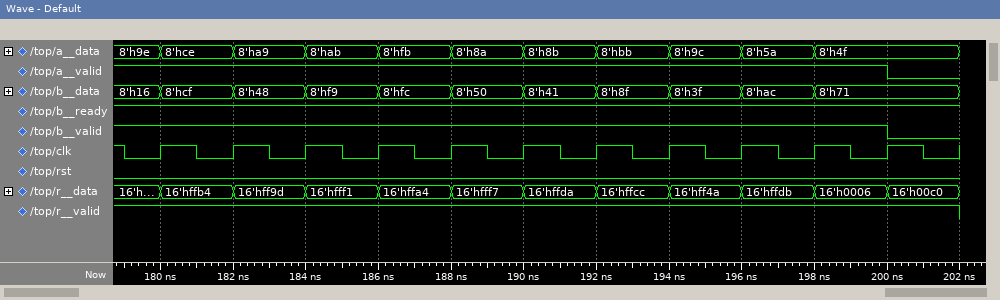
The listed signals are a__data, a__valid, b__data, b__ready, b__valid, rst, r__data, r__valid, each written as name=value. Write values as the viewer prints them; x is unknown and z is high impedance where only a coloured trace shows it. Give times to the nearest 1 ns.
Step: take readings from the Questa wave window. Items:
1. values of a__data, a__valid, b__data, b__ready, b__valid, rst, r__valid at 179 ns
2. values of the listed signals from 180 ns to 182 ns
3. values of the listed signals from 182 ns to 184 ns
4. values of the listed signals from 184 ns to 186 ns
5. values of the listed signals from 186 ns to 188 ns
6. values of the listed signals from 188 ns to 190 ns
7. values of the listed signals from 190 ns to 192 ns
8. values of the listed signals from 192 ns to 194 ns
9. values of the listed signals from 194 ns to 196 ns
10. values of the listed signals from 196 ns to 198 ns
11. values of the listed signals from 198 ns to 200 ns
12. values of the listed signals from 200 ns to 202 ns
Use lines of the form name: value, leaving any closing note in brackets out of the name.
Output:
values of a__data, a__valid, b__data, b__ready, b__valid, rst, r__valid at 179 ns: a__data=8'h9e, a__valid=1, b__data=8'h16, b__ready=1, b__valid=1, rst=0, r__valid=1
values of the listed signals from 180 ns to 182 ns: a__data=8'hce, a__valid=1, b__data=8'hcf, b__ready=1, b__valid=1, rst=0, r__data=16'hffb4, r__valid=1
values of the listed signals from 182 ns to 184 ns: a__data=8'ha9, a__valid=1, b__data=8'h48, b__ready=1, b__valid=1, rst=0, r__data=16'hff9d, r__valid=1
values of the listed signals from 184 ns to 186 ns: a__data=8'hab, a__valid=1, b__data=8'hf9, b__ready=1, b__valid=1, rst=0, r__data=16'hfff1, r__valid=1
values of the listed signals from 186 ns to 188 ns: a__data=8'hfb, a__valid=1, b__data=8'hfc, b__ready=1, b__valid=1, rst=0, r__data=16'hffa4, r__valid=1
values of the listed signals from 188 ns to 190 ns: a__data=8'h8a, a__valid=1, b__data=8'h50, b__ready=1, b__valid=1, rst=0, r__data=16'hfff7, r__valid=1
values of the listed signals from 190 ns to 192 ns: a__data=8'h8b, a__valid=1, b__data=8'h41, b__ready=1, b__valid=1, rst=0, r__data=16'hffda, r__valid=1
values of the listed signals from 192 ns to 194 ns: a__data=8'hbb, a__valid=1, b__data=8'h8f, b__ready=1, b__valid=1, rst=0, r__data=16'hffcc, r__valid=1
values of the listed signals from 194 ns to 196 ns: a__data=8'h9c, a__valid=1, b__data=8'h3f, b__ready=1, b__valid=1, rst=0, r__data=16'hff4a, r__valid=1
values of the listed signals from 196 ns to 198 ns: a__data=8'h5a, a__valid=1, b__data=8'hac, b__ready=1, b__valid=1, rst=0, r__data=16'hffdb, r__valid=1
values of the listed signals from 198 ns to 200 ns: a__data=8'h4f, a__valid=1, b__data=8'h71, b__ready=1, b__valid=1, rst=0, r__data=16'h0006, r__valid=1
values of the listed signals from 200 ns to 202 ns: a__data=8'h4f, a__valid=0, b__data=8'h71, b__ready=1, b__valid=0, rst=0, r__data=16'h00c0, r__valid=1
